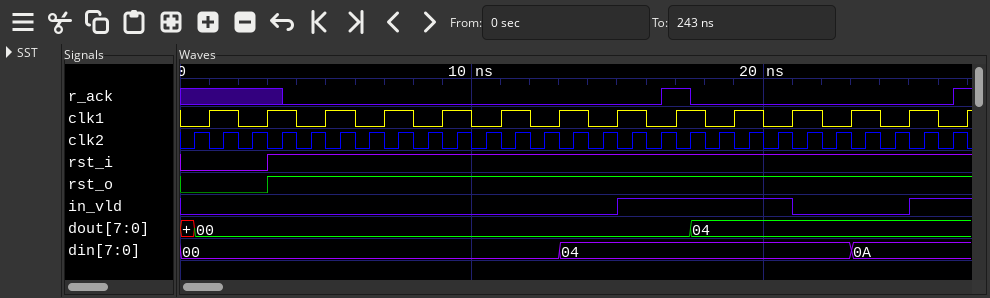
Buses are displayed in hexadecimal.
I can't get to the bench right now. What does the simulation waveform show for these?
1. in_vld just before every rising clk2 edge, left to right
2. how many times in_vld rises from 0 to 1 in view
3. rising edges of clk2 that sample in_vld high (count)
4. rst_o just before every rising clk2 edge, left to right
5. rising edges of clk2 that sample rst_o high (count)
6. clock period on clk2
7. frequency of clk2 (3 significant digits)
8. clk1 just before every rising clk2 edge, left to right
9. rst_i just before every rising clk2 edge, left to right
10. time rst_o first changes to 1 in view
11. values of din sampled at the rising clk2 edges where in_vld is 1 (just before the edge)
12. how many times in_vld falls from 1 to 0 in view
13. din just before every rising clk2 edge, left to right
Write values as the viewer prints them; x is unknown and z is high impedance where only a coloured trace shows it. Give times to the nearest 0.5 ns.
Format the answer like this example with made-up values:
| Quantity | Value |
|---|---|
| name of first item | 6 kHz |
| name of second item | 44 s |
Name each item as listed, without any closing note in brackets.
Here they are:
| Quantity | Value |
|---|---|
| in_vld just before every rising clk2 edge, left to right | 0 0 0 0 0 0 0 0 0 0 0 0 0 0 0 1 1 1 1 1 1 0 0 0 0 1 1 |
| how many times in_vld rises from 0 to 1 in view | 2 |
| rising edges of clk2 that sample in_vld high | 8 |
| rst_o just before every rising clk2 edge, left to right | 0 0 0 1 1 1 1 1 1 1 1 1 1 1 1 1 1 1 1 1 1 1 1 1 1 1 1 |
| rising edges of clk2 that sample rst_o high | 24 |
| clock period on clk2 | 1 ns |
| frequency of clk2 | 1.00 GHz |
| clk1 just before every rising clk2 edge, left to right | 0 1 0 1 0 1 0 1 0 1 0 1 0 1 0 1 0 1 0 1 0 1 0 1 0 1 0 |
| rst_i just before every rising clk2 edge, left to right | 0 0 0 1 1 1 1 1 1 1 1 1 1 1 1 1 1 1 1 1 1 1 1 1 1 1 1 |
| time rst_o first changes to 1 in view | 3 ns |
| values of din sampled at the rising clk2 edges where in_vld is 1 | 04, 04, 04, 04, 04, 04, 0A, 0A |
| how many times in_vld falls from 1 to 0 in view | 1 |
| din just before every rising clk2 edge, left to right | 00, 00, 00, 00, 00, 00, 00, 00, 00, 00, 00, 00, 00, 04, 04, 04, 04, 04, 04, 04, 04, 04, 04, 0A, 0A, 0A, 0A |
